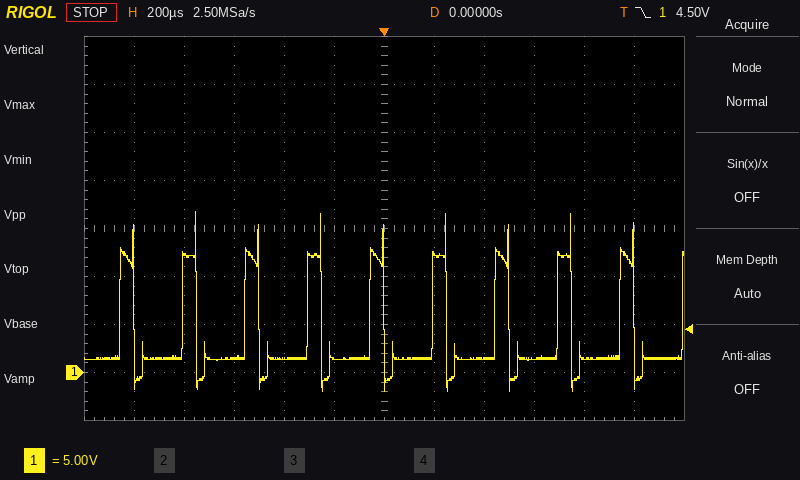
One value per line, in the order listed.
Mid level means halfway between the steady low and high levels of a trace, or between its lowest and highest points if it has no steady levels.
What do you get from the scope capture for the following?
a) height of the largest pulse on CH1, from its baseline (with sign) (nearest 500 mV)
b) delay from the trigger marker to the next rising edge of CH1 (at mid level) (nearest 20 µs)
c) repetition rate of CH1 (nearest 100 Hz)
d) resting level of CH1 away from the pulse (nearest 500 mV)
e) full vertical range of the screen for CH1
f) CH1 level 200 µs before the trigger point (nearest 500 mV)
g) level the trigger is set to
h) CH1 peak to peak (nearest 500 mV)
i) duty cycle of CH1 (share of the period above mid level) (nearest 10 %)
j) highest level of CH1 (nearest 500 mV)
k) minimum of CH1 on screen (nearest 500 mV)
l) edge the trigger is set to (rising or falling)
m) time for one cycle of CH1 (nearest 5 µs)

+15.5 V
200 µs
4.0 kHz
1.5 V
40 V
1.5 V
4.50 V
19.0 V
20 %
17.0 V
-2.0 V
falling
250 µs
